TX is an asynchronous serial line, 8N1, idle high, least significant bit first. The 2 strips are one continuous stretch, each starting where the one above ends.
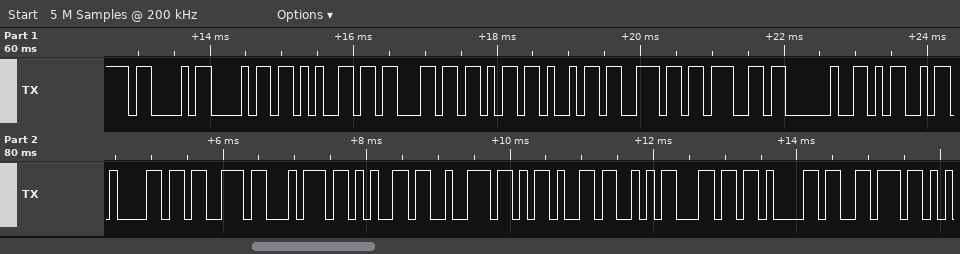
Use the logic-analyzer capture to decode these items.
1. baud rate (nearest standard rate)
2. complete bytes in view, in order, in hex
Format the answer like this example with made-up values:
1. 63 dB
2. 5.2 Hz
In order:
1. 9600 baud
2. 0x43 0x68 0x65 0x63 0x6B 0x69 0x6E 0x67 0x20 0x4D 0x61 0x73 0x74 0x65 0x72 0x2D 0x53 0x6C 0x61 0x76
